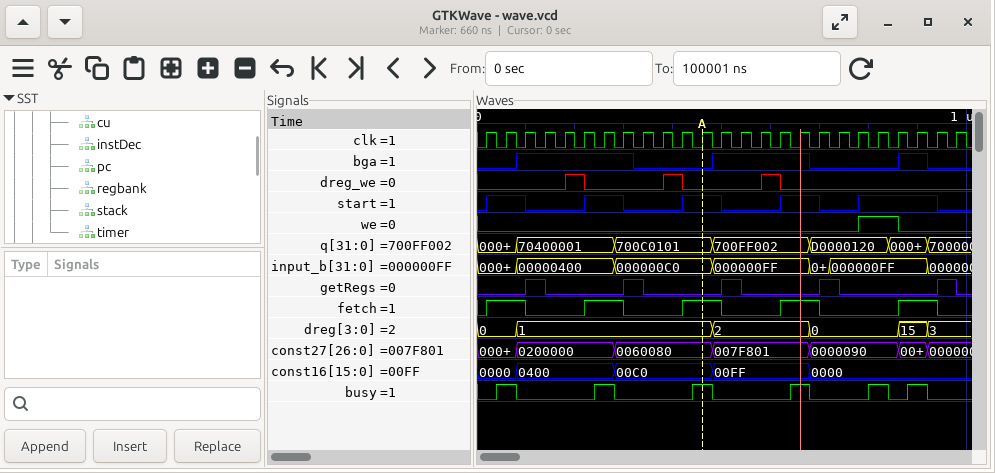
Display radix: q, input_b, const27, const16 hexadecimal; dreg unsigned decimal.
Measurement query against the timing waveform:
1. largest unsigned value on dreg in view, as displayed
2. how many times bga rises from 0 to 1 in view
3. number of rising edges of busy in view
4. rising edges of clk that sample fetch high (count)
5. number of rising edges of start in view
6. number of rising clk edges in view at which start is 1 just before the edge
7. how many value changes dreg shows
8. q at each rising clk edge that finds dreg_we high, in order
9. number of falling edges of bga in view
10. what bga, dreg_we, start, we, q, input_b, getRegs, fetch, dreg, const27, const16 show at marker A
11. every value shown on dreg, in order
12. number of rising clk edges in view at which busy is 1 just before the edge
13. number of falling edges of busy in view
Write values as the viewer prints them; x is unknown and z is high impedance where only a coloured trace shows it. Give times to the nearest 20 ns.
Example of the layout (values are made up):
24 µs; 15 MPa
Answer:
15; 3; 6; 10; 5; 12; 5; 70400001, 700C0101, 700FF002; 3; bga=0, dreg_we=0, start=1, we=0, q=700C0101, input_b=000000C0, getRegs=0, fetch=1, dreg=1, const27=0060080, const16=00C0; 0, 1, 2, 0, 15, 3; 6; 6
